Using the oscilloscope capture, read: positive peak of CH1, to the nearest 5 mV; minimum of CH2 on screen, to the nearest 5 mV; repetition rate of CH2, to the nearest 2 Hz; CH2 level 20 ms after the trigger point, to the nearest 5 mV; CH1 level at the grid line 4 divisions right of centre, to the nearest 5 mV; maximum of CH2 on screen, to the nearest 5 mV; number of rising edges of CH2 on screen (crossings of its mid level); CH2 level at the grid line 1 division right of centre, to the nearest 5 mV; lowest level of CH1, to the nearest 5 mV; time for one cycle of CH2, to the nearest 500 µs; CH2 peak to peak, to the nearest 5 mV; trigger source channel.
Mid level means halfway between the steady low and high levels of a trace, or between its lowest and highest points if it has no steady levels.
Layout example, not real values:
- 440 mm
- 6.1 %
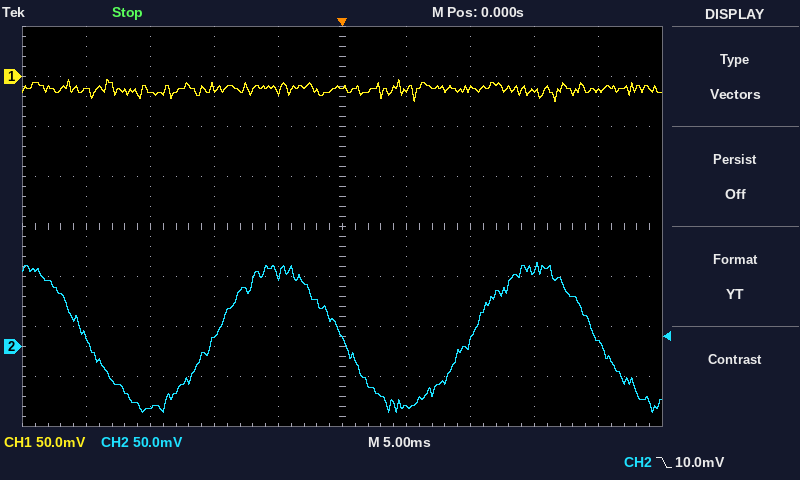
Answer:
- -5 mV
- -65 mV
- 50 Hz
- 5 mV
- -15 mV
- 85 mV
- 2
- -60 mV
- -25 mV
- 20.0 ms
- 150 mV
- CH2
